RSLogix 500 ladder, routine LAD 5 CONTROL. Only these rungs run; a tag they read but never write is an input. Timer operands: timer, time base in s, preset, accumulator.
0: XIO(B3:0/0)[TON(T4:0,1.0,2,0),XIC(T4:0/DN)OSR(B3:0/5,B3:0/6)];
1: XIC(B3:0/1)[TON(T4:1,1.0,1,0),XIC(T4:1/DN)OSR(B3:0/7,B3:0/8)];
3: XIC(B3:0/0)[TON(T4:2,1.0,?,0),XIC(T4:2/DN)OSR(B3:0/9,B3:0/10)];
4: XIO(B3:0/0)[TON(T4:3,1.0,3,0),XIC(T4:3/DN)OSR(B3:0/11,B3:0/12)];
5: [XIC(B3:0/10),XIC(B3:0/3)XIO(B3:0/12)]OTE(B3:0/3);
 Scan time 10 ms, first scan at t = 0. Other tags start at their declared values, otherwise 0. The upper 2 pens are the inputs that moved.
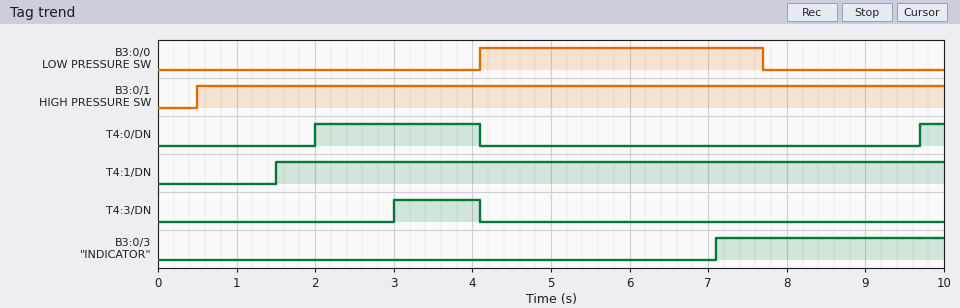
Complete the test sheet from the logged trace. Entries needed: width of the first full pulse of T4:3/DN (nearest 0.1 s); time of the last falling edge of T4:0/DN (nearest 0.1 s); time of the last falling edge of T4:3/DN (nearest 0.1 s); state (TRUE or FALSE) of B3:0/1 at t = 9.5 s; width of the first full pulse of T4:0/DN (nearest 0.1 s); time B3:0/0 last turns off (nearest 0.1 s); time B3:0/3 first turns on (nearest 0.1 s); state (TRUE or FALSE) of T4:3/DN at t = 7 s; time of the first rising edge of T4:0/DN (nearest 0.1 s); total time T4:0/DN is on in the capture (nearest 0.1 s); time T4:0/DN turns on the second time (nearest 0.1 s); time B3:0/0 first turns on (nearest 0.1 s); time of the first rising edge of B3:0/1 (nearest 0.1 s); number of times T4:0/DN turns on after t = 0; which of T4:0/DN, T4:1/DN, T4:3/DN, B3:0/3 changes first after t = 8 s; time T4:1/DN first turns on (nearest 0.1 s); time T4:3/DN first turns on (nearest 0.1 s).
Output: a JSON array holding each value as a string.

["1.1 s", "4.1 s", "4.1 s", "TRUE", "2.1 s", "7.7 s", "7.1 s", "FALSE", "2.0 s", "2.4 s", "9.7 s", "4.1 s", "0.5 s", "2", "T4:0/DN", "1.5 s", "3.0 s"]
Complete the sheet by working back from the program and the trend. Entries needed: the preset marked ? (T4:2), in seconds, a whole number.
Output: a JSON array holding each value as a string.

["3 s"]
